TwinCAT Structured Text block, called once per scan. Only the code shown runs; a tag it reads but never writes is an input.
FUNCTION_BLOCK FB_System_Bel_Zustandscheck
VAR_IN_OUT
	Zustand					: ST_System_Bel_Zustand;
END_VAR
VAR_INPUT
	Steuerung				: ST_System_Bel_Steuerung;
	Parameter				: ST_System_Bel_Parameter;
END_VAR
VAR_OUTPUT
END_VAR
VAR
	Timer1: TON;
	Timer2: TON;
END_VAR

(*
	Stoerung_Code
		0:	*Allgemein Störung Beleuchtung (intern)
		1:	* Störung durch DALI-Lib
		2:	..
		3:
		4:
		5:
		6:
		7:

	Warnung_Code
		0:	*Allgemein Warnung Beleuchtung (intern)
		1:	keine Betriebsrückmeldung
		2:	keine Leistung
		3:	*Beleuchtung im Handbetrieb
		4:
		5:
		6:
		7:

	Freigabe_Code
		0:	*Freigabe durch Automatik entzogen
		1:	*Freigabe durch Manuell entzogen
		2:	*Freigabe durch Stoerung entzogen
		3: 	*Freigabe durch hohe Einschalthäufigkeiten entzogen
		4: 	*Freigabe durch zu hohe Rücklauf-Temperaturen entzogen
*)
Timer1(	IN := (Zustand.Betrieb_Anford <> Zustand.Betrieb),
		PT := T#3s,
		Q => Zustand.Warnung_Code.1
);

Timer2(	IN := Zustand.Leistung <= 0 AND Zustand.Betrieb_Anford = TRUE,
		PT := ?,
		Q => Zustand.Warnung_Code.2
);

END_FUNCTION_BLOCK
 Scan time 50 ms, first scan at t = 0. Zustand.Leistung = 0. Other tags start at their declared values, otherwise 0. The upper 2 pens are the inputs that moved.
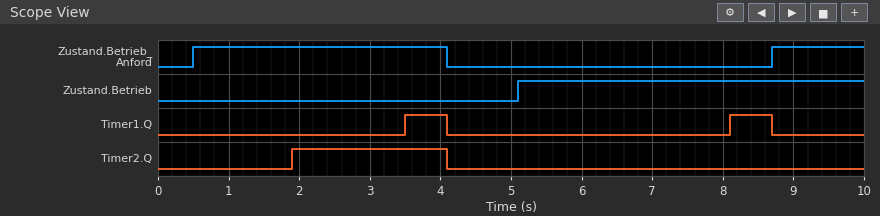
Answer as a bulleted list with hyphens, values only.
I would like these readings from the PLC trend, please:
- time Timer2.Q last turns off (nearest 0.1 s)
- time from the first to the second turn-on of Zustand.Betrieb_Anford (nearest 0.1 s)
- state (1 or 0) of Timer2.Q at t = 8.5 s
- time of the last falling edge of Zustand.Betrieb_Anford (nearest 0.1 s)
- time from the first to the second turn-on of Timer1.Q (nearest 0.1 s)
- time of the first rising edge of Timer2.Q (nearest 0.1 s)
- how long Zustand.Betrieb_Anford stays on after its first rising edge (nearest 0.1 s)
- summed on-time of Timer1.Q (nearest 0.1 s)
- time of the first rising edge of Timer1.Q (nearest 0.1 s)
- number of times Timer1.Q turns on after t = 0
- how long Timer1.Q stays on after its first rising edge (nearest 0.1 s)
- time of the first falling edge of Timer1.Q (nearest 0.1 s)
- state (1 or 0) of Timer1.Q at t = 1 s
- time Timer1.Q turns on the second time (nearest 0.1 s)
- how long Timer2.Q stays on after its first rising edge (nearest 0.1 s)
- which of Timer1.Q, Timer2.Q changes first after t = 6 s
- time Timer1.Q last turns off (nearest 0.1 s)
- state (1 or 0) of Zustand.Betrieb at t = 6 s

- 4.1 s
- 8.2 s
- 0
- 4.1 s
- 4.6 s
- 1.9 s
- 3.6 s
- 1.2 s
- 3.5 s
- 2
- 0.6 s
- 4.1 s
- 0
- 8.1 s
- 2.2 s
- Timer1.Q
- 8.7 s
- 1
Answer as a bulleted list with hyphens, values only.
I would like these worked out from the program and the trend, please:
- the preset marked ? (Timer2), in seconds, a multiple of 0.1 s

- 1.4 s
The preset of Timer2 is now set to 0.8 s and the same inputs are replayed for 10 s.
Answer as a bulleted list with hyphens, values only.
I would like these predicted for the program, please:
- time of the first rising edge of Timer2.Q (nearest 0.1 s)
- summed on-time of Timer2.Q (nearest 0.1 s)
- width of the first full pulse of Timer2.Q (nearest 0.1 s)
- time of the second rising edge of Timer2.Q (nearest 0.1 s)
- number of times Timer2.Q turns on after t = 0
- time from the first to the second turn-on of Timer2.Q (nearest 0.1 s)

- 1.3 s
- 3.3 s
- 2.8 s
- 9.5 s
- 2
- 8.2 s
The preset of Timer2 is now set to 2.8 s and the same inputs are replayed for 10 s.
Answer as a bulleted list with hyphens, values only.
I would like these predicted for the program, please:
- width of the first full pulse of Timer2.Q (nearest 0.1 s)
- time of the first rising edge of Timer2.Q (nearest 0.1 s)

- 0.8 s
- 3.3 s
